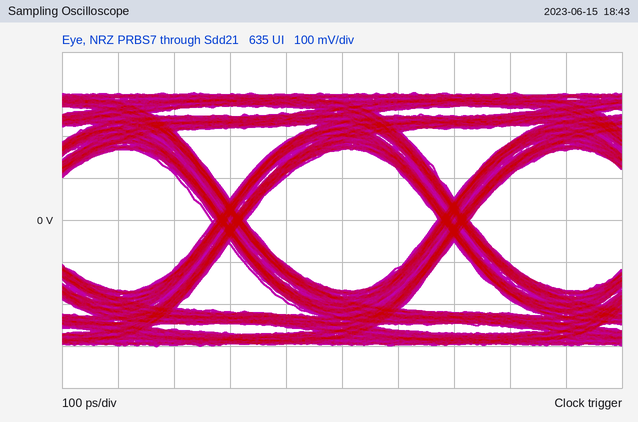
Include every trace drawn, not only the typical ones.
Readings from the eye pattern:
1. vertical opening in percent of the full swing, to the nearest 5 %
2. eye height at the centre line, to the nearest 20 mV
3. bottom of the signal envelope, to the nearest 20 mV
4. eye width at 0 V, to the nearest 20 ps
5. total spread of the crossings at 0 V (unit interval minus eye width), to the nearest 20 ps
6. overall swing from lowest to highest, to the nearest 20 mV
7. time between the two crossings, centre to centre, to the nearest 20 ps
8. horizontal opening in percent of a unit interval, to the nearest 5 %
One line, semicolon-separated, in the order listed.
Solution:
55 %; 340 mV; -300 mV; 340 ps; 60 ps; 600 mV; 400 ps; 85 %
